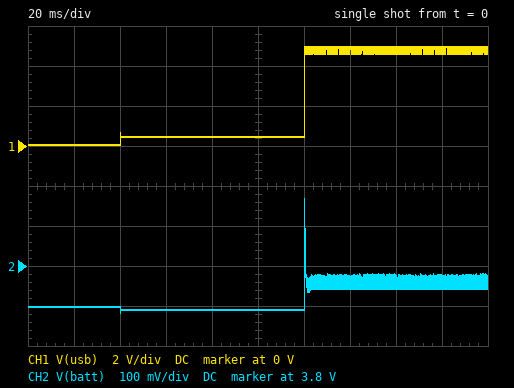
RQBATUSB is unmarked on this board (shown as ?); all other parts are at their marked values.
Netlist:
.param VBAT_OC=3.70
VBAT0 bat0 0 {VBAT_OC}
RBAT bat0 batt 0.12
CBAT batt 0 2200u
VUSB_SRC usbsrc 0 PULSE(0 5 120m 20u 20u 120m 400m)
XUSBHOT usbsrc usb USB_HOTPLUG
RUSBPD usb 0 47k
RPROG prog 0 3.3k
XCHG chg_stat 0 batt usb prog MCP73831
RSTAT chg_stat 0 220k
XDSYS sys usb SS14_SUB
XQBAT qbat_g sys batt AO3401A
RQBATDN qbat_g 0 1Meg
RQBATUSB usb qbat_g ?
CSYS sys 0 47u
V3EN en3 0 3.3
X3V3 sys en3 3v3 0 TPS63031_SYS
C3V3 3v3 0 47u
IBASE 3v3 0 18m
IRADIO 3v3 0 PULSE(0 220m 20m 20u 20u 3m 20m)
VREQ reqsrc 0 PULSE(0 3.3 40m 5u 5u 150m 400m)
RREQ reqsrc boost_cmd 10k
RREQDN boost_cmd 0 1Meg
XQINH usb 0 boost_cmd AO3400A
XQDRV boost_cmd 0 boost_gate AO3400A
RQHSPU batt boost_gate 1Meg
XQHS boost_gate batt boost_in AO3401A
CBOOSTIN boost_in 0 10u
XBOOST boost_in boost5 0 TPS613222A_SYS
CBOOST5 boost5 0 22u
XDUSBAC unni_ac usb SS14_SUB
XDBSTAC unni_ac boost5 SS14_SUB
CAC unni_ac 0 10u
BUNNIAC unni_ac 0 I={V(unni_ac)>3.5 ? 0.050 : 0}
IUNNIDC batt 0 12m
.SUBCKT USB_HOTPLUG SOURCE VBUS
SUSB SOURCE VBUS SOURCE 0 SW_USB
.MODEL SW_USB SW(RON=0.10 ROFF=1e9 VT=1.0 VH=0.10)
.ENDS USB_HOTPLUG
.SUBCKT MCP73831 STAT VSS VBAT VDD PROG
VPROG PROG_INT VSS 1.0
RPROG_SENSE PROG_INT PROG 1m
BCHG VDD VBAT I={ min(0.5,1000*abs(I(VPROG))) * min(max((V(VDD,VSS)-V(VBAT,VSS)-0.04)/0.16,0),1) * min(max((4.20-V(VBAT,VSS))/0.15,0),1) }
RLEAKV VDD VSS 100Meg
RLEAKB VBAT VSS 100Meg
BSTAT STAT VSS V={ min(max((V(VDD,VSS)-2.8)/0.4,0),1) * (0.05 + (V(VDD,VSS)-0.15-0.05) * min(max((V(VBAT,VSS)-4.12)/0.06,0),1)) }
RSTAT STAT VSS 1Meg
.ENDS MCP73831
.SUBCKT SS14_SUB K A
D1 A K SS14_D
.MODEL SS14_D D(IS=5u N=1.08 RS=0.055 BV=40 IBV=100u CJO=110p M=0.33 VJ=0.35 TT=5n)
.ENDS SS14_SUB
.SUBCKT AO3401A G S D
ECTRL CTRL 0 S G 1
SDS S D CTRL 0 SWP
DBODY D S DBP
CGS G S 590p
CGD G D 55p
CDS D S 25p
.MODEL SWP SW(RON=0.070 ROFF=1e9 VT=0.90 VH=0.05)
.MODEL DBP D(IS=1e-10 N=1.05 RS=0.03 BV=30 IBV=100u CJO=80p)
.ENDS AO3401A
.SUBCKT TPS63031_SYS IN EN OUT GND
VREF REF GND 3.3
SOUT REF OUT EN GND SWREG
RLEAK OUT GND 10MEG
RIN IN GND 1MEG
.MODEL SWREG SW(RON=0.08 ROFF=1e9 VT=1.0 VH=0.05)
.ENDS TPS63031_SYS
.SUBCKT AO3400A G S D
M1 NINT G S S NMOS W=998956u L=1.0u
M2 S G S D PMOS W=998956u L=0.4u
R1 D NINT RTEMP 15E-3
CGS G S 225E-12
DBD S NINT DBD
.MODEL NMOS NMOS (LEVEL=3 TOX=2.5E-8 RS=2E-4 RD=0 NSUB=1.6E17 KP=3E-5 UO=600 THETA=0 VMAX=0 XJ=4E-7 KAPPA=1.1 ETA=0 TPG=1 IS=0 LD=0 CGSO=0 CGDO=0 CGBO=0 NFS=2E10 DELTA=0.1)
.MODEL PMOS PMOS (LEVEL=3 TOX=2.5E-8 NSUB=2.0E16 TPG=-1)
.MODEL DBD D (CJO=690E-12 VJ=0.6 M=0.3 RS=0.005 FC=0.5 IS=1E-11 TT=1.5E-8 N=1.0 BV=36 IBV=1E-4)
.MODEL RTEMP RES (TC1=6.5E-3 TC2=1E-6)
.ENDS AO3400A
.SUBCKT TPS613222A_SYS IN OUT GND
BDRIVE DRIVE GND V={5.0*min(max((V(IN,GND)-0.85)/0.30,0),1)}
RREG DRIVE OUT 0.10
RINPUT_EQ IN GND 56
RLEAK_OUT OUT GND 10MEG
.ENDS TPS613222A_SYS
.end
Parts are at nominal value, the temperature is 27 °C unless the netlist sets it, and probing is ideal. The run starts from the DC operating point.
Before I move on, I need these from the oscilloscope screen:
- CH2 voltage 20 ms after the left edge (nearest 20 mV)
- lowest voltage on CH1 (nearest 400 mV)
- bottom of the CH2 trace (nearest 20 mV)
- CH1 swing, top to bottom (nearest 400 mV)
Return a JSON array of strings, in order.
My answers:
["3.70 V", "0 V", "3.68 V", "4.8 V"]
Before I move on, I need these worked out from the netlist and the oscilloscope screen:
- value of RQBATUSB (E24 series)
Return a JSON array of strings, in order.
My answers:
["300 kΩ"]
